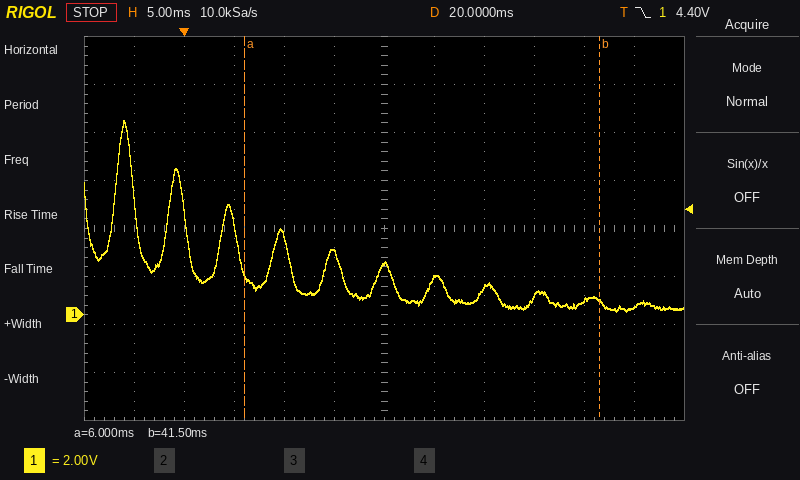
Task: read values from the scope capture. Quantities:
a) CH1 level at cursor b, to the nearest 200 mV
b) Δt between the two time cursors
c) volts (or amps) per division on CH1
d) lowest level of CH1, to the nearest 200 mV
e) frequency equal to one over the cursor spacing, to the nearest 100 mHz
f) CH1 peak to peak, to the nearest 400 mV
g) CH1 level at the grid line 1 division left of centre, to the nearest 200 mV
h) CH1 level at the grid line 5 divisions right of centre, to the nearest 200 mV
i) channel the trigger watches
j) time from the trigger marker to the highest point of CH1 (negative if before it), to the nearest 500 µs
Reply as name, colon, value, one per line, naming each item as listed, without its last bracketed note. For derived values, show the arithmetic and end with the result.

CH1 level at cursor b, to the nearest 200 mV: 600 mV
Δt between the two time cursors: 41.5 ms − (6 ms) = 35.5 ms
volts (or amps) per division on CH1: 2 V
lowest level of CH1, to the nearest 200 mV: 200 mV
frequency equal to one over the cursor spacing, to the nearest 100 mHz: 1 / 35.5 ms ≈ 28.2 Hz
CH1 peak to peak, to the nearest 400 mV: 8.0 V
CH1 level at the grid line 1 division left of centre, to the nearest 200 mV: 2.6 V
CH1 level at the grid line 5 divisions right of centre, to the nearest 200 mV: 400 mV
channel the trigger watches: CH1
time from the trigger marker to the highest point of CH1 (negative if before it), to the nearest 500 µs: -6.0 ms
